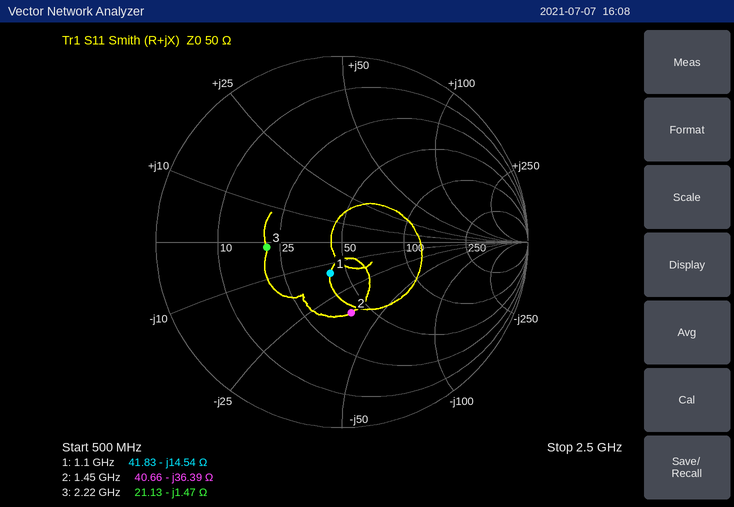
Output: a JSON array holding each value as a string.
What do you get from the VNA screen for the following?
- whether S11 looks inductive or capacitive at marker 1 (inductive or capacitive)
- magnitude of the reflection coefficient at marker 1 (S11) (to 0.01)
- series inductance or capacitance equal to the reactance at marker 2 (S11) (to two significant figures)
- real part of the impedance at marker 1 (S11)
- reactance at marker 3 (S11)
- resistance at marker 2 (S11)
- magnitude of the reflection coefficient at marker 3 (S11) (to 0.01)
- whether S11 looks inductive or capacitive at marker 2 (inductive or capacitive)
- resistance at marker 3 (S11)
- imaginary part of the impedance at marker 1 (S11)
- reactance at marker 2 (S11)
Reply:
["capacitive", "0.18", "3.0 pF", "41.83 Ω", "-1.47 Ω", "40.66 Ω", "0.41", "capacitive", "21.13 Ω", "-14.54 Ω", "-36.39 Ω"]
